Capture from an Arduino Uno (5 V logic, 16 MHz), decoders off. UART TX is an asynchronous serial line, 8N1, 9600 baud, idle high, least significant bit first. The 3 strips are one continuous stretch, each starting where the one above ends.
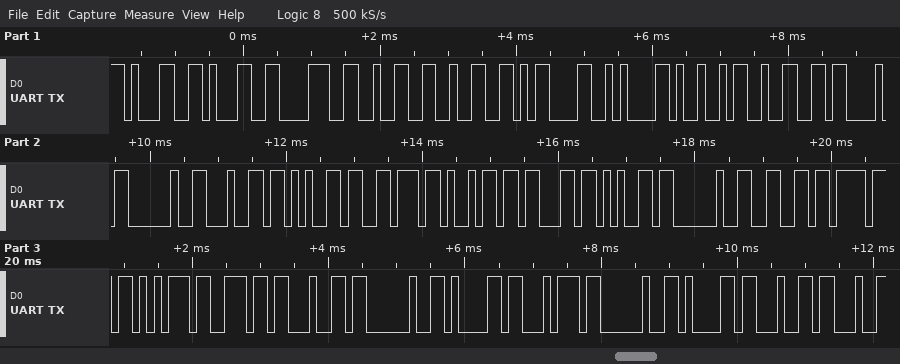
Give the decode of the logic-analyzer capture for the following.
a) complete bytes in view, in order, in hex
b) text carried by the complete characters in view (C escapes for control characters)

31 31 38 32 32 0D 0A 49 32 43 20 64 65 76 69 63 65 20 66 6F 75 6E 64 20 61 74 20 61 64
"11822\r\nI2C device found at ad"
